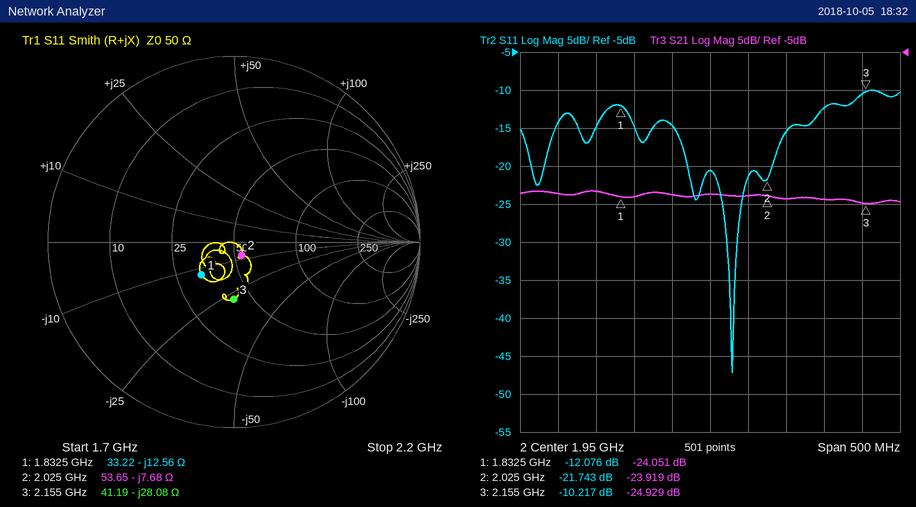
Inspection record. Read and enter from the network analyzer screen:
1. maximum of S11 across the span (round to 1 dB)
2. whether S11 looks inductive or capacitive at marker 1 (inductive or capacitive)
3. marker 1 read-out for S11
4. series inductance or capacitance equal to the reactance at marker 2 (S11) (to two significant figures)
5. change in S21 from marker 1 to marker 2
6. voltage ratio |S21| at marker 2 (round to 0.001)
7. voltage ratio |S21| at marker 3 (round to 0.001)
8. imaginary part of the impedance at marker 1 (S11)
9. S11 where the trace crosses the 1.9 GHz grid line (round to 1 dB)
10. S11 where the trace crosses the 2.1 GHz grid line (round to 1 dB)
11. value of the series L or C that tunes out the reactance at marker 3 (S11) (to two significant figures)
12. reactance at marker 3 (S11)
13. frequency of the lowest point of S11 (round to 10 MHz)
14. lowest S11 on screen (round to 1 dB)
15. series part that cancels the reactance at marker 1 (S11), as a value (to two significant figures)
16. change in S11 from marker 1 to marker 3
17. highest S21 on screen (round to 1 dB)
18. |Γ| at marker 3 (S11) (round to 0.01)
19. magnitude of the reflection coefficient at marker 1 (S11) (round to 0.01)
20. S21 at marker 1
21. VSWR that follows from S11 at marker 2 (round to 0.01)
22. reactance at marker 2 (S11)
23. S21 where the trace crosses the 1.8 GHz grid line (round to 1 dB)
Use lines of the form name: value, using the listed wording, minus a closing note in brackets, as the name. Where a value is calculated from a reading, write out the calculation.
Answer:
maximum of S11 across the span: -10 dB
whether S11 looks inductive or capacitive at marker 1: capacitive
marker 1 read-out for S11: -12.076 dB
series inductance or capacitance equal to the reactance at marker 2 (S11): C = 1/(2π × 2.025 GHz × 7.68 Ω) ≈ 10 pF
change in S21 from marker 1 to marker 2: -23.919 − (-24.051) = 0.132 dB
voltage ratio |S21| at marker 2: 10^(-23.919/20) ≈ 0.064
voltage ratio |S21| at marker 3: 10^(-24.929/20) ≈ 0.057
imaginary part of the impedance at marker 1: -12.56 Ω
S11 where the trace crosses the 1.9 GHz grid line: -15 dB
S11 where the trace crosses the 2.1 GHz grid line: -12 dB
value of the series L or C that tunes out the reactance at marker 3 (S11): L = 28.08 Ω/(2π × 2.155 GHz) ≈ 2.1 nH
reactance at marker 3: -28.08 Ω
frequency of the lowest point of S11: 1.98 GHz
lowest S11 on screen: -47 dB
series part that cancels the reactance at marker 1 (S11), as a value: L = 12.56 Ω/(2π × 1.8325 GHz) ≈ 1.1 nH
change in S11 from marker 1 to marker 3: -10.217 − (-12.076) = 1.859 dB
highest S21 on screen: -23 dB
|Γ| at marker 3 (S11): 0.31
magnitude of the reflection coefficient at marker 1 (S11): 0.25
S21 at marker 1: -24.051 dB
VSWR that follows from S11 at marker 2: (1 + 0.0818)/(1 − 0.0818) ≈ 1.18
reactance at marker 2: -7.68 Ω
S21 where the trace crosses the 1.8 GHz grid line: -23 dB
